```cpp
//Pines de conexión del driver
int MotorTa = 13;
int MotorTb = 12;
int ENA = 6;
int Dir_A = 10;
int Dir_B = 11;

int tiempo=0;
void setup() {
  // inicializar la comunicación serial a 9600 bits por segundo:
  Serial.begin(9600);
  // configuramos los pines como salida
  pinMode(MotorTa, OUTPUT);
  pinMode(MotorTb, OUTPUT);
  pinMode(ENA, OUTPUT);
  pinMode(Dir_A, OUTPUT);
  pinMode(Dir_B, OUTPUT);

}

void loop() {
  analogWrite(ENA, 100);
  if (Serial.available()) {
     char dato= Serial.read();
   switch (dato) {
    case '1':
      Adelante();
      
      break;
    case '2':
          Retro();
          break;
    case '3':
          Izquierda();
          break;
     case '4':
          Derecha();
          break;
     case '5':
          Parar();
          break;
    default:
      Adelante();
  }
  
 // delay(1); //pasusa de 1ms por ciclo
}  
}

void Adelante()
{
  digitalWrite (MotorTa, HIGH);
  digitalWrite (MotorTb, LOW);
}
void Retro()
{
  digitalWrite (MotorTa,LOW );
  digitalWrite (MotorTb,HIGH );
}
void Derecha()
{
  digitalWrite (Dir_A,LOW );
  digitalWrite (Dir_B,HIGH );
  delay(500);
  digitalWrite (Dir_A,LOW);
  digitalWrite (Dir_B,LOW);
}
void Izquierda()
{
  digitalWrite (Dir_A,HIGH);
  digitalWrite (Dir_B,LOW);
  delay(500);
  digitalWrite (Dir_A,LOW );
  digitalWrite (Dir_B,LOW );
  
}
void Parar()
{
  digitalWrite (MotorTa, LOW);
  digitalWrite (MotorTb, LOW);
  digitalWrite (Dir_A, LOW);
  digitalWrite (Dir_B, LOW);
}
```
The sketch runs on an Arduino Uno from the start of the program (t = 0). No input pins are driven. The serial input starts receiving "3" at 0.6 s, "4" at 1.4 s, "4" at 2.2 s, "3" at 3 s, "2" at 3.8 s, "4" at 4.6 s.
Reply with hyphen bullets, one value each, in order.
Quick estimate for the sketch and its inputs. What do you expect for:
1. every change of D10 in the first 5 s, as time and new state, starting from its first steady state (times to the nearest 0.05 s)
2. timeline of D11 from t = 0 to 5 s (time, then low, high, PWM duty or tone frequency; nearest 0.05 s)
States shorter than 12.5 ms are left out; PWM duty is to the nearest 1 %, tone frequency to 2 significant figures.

- 0 s low; 0.6 s high; 1.1 s low; 3 s high; 3.5 s low
- 0 s low; 1.4 s high; 1.9 s low; 2.2 s high; 2.7 s low; 4.6 s high
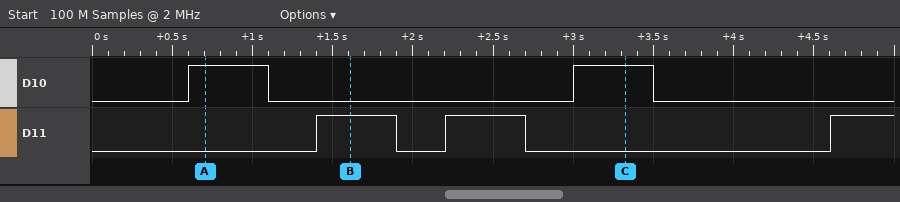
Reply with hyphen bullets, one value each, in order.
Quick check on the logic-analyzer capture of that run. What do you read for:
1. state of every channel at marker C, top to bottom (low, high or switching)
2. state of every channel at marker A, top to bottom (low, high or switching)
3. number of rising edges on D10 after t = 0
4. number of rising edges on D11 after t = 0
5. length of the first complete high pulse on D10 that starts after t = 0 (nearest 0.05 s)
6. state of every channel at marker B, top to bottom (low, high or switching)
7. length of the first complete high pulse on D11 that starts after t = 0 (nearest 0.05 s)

- D10 high, D11 low
- D10 high, D11 low
- 2
- 3
- 0.50 s
- D10 low, D11 high
- 0.50 s
